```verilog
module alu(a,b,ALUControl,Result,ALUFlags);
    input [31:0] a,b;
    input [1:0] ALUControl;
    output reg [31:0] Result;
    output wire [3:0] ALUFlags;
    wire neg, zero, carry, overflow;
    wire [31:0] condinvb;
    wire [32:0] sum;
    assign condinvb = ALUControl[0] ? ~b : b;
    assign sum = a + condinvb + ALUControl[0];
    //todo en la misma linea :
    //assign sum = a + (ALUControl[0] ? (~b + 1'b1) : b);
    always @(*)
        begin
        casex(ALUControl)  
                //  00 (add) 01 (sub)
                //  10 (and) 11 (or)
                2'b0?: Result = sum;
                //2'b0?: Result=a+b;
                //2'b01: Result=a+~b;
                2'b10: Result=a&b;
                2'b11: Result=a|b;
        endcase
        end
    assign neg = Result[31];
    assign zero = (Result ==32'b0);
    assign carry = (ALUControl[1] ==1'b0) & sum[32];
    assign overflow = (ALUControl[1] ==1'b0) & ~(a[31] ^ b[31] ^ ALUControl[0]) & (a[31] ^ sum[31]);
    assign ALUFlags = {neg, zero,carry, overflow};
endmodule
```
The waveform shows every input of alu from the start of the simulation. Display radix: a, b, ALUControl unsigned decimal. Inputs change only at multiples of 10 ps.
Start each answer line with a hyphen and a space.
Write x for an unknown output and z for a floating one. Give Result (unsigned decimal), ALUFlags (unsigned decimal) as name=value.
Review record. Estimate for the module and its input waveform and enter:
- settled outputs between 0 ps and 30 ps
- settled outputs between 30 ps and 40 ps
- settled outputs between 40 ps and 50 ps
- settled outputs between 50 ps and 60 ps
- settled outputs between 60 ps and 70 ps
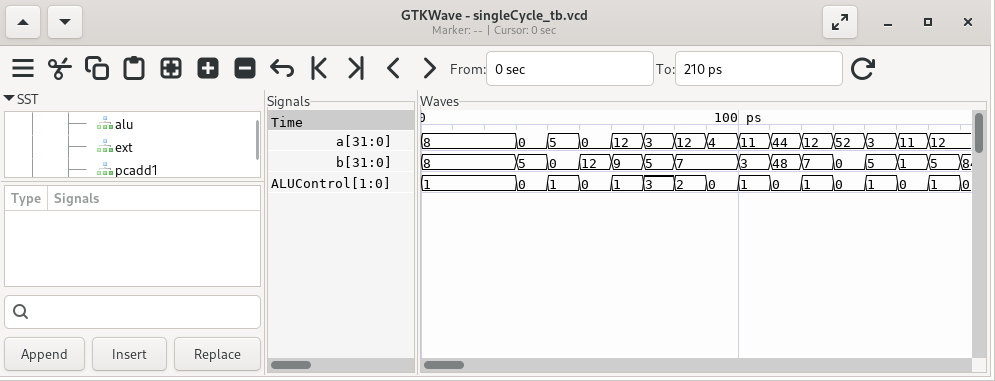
- Result=0, ALUFlags=6
- Result=5, ALUFlags=0
- Result=5, ALUFlags=2
- Result=12, ALUFlags=0
- Result=3, ALUFlags=2
